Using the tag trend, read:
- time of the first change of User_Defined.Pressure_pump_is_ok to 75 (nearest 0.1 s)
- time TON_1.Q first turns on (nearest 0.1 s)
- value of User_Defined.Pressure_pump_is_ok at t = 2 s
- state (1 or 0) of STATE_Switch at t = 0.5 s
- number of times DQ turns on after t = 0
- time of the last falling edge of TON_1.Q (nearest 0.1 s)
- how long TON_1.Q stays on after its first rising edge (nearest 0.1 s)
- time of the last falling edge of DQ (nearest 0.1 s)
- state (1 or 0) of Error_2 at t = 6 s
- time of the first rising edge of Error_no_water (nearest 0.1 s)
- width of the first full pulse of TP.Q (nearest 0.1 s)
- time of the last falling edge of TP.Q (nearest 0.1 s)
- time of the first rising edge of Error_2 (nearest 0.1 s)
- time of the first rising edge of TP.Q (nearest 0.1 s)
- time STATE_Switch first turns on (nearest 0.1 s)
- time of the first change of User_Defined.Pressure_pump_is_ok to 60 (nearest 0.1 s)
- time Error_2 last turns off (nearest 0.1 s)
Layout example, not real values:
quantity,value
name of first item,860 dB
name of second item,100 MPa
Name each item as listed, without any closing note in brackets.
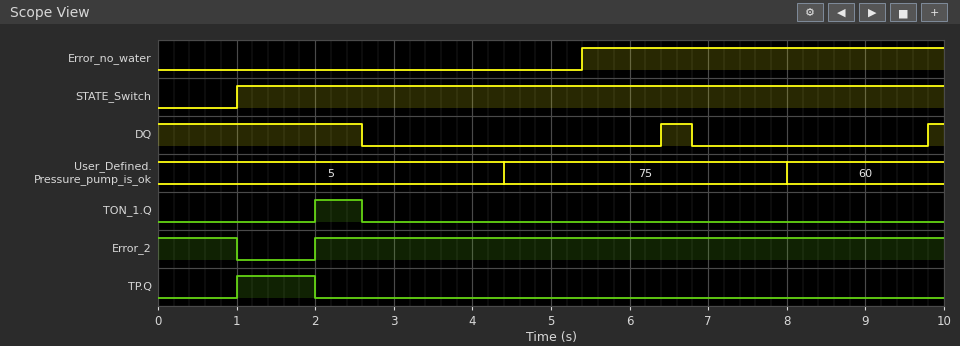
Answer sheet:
quantity,value
time of the first change of User_Defined.Pressure_pump_is_ok to 75,4.4 s
time TON_1.Q first turns on,2.0 s
value of User_Defined.Pressure_pump_is_ok at t = 2 s,5
state (1 or 0) of STATE_Switch at t = 0.5 s,0
number of times DQ turns on after t = 0,2
time of the last falling edge of TON_1.Q,2.6 s
how long TON_1.Q stays on after its first rising edge,0.6 s
time of the last falling edge of DQ,6.8 s
state (1 or 0) of Error_2 at t = 6 s,1
time of the first rising edge of Error_no_water,5.4 s
width of the first full pulse of TP.Q,1.0 s
time of the last falling edge of TP.Q,2.0 s
time of the first rising edge of Error_2,2.0 s
time of the first rising edge of TP.Q,1.0 s
time STATE_Switch first turns on,1.0 s
time of the first change of User_Defined.Pressure_pump_is_ok to 60,8.0 s
time Error_2 last turns off,1.0 s
